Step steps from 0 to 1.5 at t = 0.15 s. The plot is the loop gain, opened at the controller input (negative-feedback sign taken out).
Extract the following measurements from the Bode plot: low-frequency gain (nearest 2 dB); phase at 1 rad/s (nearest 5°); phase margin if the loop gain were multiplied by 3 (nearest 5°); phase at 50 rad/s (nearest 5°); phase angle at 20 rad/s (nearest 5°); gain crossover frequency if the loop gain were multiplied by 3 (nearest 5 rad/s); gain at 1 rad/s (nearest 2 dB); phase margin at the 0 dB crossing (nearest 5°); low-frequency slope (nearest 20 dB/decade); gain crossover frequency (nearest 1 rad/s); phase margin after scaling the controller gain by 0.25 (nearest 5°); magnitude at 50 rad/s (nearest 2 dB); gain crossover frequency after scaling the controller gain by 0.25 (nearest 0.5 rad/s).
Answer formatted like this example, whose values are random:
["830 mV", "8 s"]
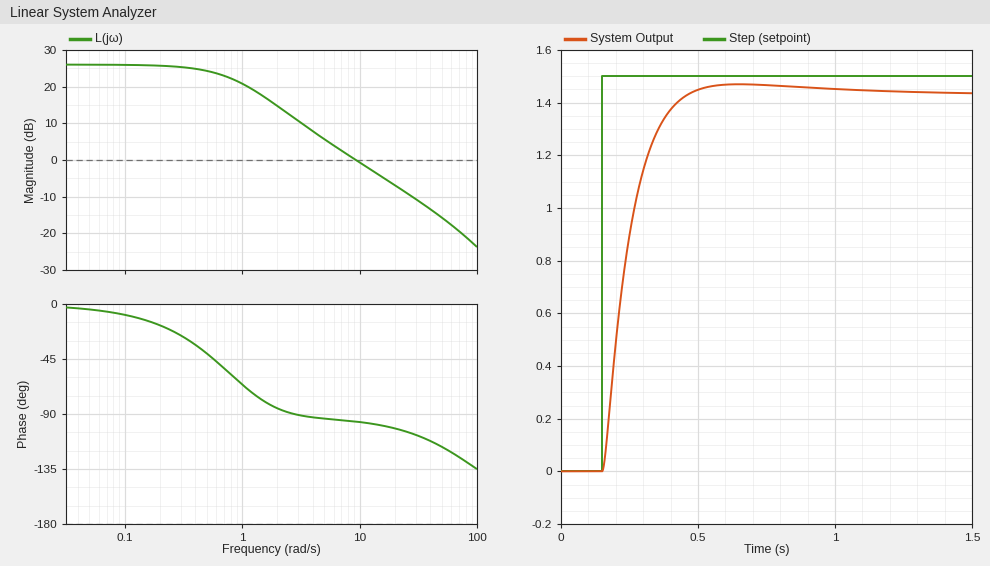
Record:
["26 dB", "-65°", "75°", "-115°", "-100°", "25 rad/s", "20 dB", "85°", "0 dB/decade", "9 rad/s", "90°", "-16 dB", "2.5 rad/s"]
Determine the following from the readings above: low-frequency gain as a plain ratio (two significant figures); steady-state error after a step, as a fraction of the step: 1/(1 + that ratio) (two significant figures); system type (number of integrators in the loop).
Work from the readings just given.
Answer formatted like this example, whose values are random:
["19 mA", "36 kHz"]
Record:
["20", "0.048", "0"]
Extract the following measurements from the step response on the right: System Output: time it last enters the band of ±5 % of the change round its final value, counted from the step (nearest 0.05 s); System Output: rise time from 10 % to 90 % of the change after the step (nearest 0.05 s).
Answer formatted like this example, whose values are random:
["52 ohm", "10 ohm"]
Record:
["0.25 s", "0.20 s"]
